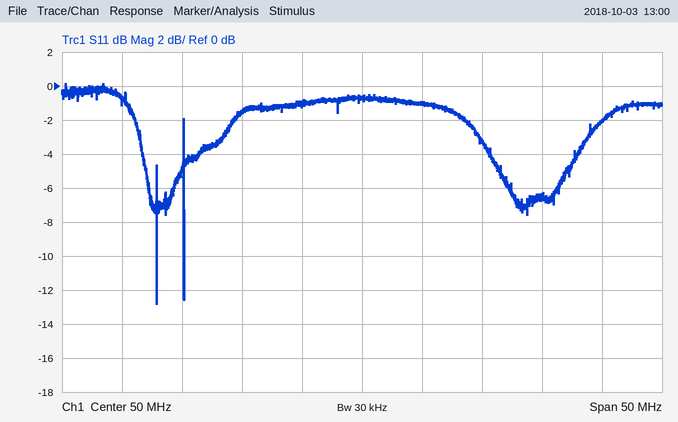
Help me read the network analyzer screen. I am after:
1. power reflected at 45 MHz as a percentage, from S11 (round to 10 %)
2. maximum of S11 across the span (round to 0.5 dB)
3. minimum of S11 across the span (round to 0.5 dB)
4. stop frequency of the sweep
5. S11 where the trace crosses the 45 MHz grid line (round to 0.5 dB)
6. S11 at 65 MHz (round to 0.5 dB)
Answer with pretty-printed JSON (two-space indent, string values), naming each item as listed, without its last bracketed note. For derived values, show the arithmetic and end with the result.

{
  "power reflected at 45 MHz as a percentage, from S11": "10^(-1/10) ≈ 79.4 %, so 80 % to the nearest 10 %",
  "maximum of S11 across the span": "0.0 dB",
  "minimum of S11 across the span": "-13.0 dB",
  "stop frequency of the sweep": "75 MHz",
  "S11 where the trace crosses the 45 MHz grid line": "-1.0 dB",
  "S11 at 65 MHz": "-6.5 dB"
}
